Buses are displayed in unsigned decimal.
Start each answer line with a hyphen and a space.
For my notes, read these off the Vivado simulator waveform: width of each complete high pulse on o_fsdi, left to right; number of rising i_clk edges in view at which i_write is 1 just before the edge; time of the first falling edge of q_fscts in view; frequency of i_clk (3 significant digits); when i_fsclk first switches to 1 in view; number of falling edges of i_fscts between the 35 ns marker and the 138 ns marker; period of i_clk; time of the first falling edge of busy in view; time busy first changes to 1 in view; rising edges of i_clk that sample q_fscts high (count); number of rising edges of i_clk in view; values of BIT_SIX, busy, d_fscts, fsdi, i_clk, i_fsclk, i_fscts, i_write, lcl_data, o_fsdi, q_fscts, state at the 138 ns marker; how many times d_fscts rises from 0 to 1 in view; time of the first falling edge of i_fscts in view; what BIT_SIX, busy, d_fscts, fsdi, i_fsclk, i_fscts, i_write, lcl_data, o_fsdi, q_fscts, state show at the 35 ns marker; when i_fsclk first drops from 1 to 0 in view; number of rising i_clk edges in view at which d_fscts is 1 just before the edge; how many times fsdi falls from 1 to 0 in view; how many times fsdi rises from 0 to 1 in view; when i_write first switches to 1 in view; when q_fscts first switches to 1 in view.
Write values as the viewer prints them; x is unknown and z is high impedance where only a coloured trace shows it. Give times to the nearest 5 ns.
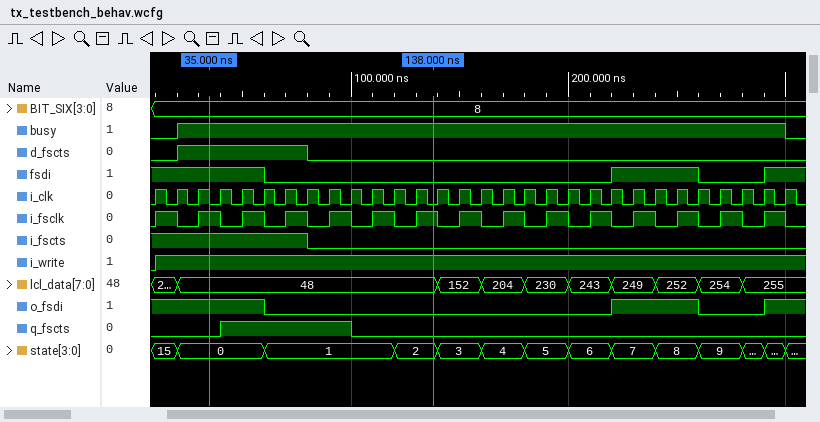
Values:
- 40 ns
- 29
- 100 ns
- 100 MHz
- 10 ns
- 1
- 10 ns
- 300 ns
- 20 ns
- 6
- 30
- BIT_SIX=8, busy=1, d_fscts=0, fsdi=0, i_clk=0, i_fsclk=1, i_fscts=0, i_write=1, lcl_data=48, o_fsdi=0, q_fscts=0, state=2
- 1
- 80 ns
- BIT_SIX=8, busy=1, d_fscts=1, fsdi=1, i_fsclk=1, i_fscts=1, i_write=1, lcl_data=48, o_fsdi=1, q_fscts=0, state=0
- 20 ns
- 6
- 2
- 2
- 10 ns
- 40 ns
